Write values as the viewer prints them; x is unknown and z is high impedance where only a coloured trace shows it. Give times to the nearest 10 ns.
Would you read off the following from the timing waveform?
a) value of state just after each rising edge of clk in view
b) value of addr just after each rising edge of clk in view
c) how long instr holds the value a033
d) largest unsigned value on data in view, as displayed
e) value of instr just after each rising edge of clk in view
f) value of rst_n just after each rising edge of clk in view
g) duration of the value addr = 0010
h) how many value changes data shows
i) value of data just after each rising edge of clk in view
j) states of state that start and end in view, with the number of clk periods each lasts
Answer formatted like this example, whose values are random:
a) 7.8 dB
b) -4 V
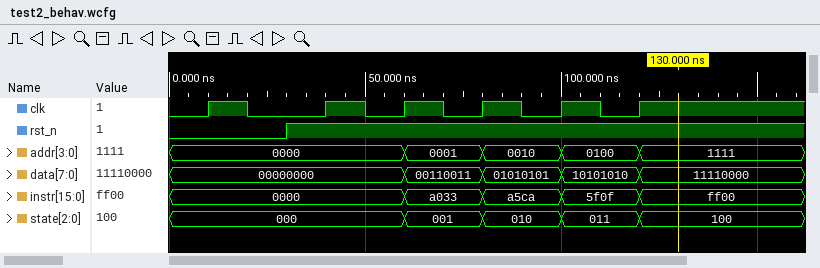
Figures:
a) 000, 000, 001, 010, 011, 100
b) 0000, 0000, 0001, 0010, 0100, 1111
c) 20 ns
d) 11110000
e) 0000, 0000, a033, a5ca, 5f0f, ff00
f) 0 1 1 1 1 1
g) 20 ns
h) 4
i) 00000000, 00000000, 00110011, 01010101, 10101010, 11110000
j) 001: 1, 010: 1, 011: 1
